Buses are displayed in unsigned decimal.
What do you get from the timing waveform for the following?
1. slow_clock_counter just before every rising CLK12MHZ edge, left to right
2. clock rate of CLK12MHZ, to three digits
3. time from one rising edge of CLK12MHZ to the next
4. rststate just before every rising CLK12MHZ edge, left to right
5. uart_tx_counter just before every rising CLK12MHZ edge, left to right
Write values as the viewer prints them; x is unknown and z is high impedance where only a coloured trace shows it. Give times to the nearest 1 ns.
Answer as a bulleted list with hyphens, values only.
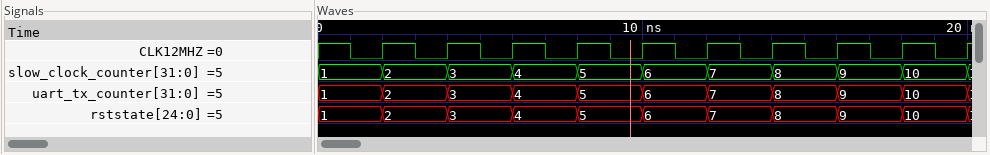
- 1, 2, 3, 4, 5, 6, 7, 8, 9, 10
- 500 MHz
- 2 ns
- 1, 2, 3, 4, 5, 6, 7, 8, 9, 10
- 1, 2, 3, 4, 5, 6, 7, 8, 9, 10
